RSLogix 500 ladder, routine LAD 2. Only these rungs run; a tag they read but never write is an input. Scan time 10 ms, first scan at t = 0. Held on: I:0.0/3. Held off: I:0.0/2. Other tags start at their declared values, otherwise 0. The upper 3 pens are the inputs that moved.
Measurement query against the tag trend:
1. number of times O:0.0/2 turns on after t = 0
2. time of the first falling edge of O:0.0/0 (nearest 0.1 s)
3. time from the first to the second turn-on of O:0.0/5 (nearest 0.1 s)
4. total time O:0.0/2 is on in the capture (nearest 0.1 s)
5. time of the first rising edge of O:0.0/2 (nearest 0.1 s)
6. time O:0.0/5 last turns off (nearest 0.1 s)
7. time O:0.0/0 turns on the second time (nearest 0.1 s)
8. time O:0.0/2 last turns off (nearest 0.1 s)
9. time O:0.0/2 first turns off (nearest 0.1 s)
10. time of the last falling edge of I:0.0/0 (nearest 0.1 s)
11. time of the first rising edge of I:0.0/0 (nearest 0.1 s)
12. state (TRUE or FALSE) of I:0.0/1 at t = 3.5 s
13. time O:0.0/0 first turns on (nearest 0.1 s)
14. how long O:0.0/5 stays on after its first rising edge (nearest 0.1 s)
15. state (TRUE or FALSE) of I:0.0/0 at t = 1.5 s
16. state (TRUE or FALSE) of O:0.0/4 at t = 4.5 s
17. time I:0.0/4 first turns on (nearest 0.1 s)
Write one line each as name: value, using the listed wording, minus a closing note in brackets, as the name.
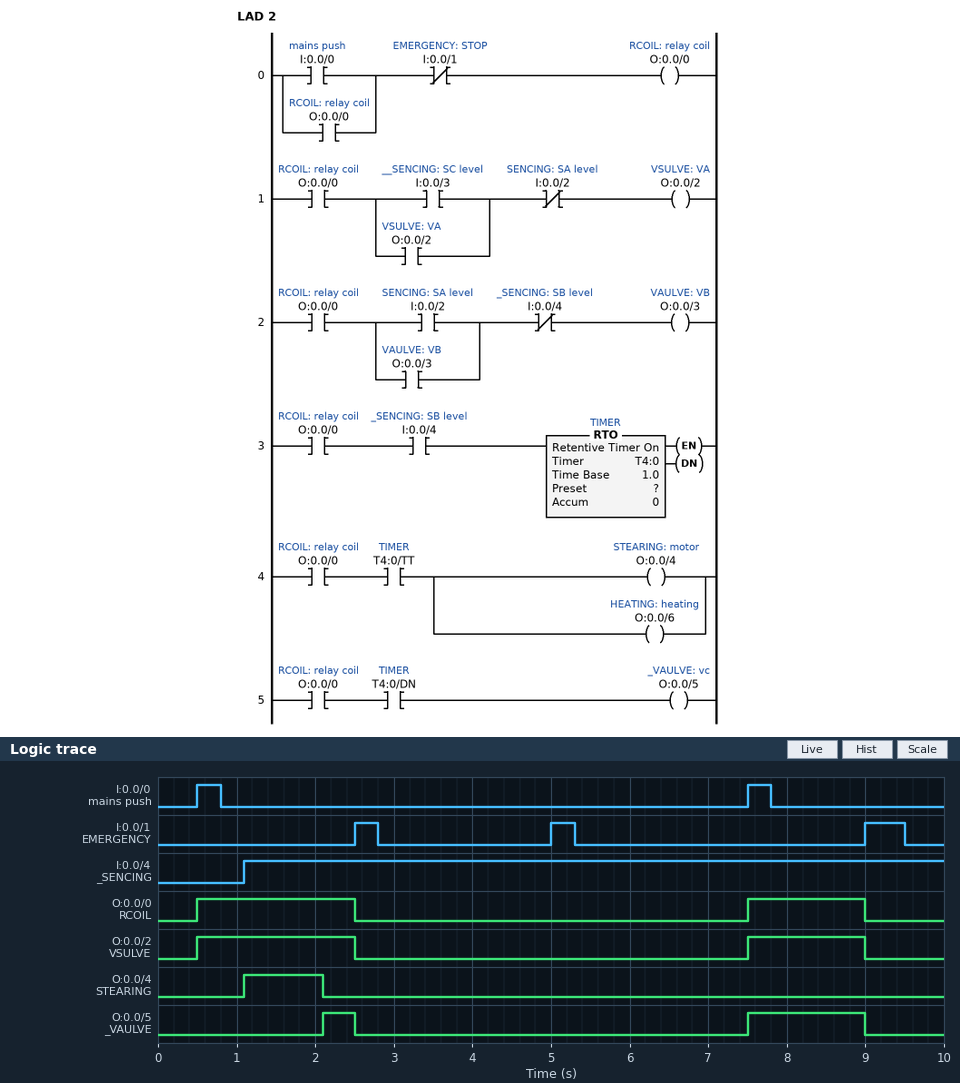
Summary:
number of times O:0.0/2 turns on after t = 0: 2
time of the first falling edge of O:0.0/0: 2.5 s
time from the first to the second turn-on of O:0.0/5: 5.4 s
total time O:0.0/2 is on in the capture: 3.5 s
time of the first rising edge of O:0.0/2: 0.5 s
time O:0.0/5 last turns off: 9.0 s
time O:0.0/0 turns on the second time: 7.5 s
time O:0.0/2 last turns off: 9.0 s
time O:0.0/2 first turns off: 2.5 s
time of the last falling edge of I:0.0/0: 7.8 s
time of the first rising edge of I:0.0/0: 0.5 s
state (TRUE or FALSE) of I:0.0/1 at t = 3.5 s: FALSE
time O:0.0/0 first turns on: 0.5 s
how long O:0.0/5 stays on after its first rising edge: 0.4 s
state (TRUE or FALSE) of I:0.0/0 at t = 1.5 s: FALSE
state (TRUE or FALSE) of O:0.0/4 at t = 4.5 s: FALSE
time I:0.0/4 first turns on: 1.1 s
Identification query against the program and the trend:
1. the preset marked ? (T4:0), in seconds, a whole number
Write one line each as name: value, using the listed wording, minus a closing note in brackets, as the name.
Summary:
the preset marked ? (T4:0), in seconds, a whole number: 1 s
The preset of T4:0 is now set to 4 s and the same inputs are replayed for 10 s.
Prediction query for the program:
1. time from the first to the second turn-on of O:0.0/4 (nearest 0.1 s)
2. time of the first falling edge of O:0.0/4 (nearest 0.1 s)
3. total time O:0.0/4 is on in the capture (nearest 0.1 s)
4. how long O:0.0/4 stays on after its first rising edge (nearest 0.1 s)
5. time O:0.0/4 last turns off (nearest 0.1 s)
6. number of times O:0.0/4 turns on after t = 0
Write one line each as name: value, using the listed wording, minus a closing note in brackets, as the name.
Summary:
time from the first to the second turn-on of O:0.0/4: 6.4 s
time of the first falling edge of O:0.0/4: 2.5 s
total time O:0.0/4 is on in the capture: 2.9 s
how long O:0.0/4 stays on after its first rising edge: 1.4 s
time O:0.0/4 last turns off: 9.0 s
number of times O:0.0/4 turns on after t = 0: 2
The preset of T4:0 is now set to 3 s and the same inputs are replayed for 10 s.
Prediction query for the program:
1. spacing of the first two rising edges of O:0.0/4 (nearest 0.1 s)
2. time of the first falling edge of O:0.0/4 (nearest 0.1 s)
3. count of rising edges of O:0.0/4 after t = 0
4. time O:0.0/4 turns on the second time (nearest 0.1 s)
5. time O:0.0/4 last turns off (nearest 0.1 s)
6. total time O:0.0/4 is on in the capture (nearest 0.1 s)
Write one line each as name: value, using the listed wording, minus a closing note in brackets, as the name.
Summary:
spacing of the first two rising edges of O:0.0/4: 6.4 s
time of the first falling edge of O:0.0/4: 2.5 s
count of rising edges of O:0.0/4 after t = 0: 2
time O:0.0/4 turns on the second time: 7.5 s
time O:0.0/4 last turns off: 9.0 s
total time O:0.0/4 is on in the capture: 2.9 s
